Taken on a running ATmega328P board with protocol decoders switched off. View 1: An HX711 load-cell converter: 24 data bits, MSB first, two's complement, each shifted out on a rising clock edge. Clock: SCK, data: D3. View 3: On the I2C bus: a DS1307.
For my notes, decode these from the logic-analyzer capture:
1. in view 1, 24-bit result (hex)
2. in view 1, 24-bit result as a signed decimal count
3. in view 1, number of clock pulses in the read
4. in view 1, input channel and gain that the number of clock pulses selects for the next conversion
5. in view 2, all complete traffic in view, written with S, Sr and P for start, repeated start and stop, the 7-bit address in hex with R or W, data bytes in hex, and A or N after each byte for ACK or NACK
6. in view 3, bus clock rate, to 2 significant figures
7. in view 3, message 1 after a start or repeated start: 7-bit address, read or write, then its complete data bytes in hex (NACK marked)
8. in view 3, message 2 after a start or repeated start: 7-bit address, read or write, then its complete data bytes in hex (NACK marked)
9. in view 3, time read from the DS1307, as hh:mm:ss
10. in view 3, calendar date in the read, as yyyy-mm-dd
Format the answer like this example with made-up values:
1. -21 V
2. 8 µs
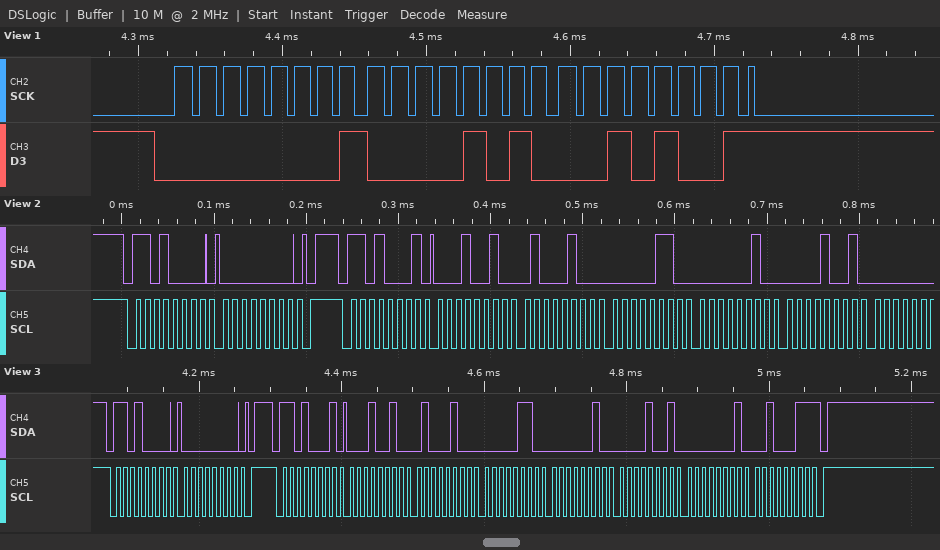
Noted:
1. 0x010A29
2. 68137
3. 25
4. channel A, gain 128
5. S 68W A 00 A P S 68R A 12 A 44 A 06 A 02 A 09 A
6. 100 kHz
7. 0x68 write: 00
8. 0x68 read: 12 44 06 02 09 01 23 NACK
9. 06:44:12
10. 2023-01-09
